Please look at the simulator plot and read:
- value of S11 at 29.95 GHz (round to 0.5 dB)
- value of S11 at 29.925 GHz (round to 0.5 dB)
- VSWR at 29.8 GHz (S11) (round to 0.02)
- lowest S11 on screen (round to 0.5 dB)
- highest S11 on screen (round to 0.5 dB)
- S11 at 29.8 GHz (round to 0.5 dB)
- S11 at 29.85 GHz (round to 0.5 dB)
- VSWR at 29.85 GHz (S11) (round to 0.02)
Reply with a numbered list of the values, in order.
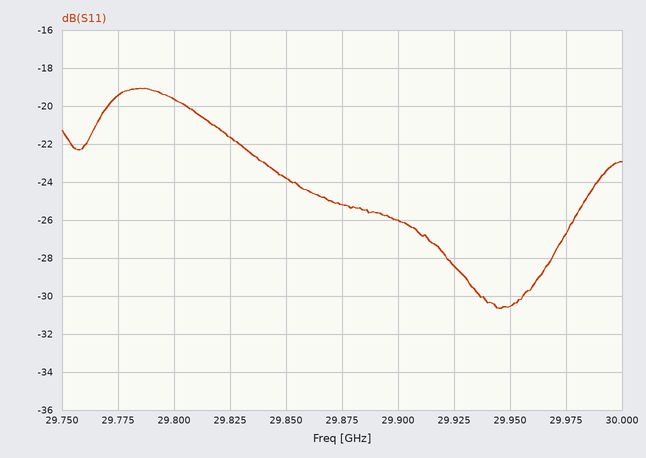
1. -30.5 dB
2. -28.5 dB
3. 1.24
4. -30.5 dB
5. -19.0 dB
6. -19.5 dB
7. -24.0 dB
8. 1.14
